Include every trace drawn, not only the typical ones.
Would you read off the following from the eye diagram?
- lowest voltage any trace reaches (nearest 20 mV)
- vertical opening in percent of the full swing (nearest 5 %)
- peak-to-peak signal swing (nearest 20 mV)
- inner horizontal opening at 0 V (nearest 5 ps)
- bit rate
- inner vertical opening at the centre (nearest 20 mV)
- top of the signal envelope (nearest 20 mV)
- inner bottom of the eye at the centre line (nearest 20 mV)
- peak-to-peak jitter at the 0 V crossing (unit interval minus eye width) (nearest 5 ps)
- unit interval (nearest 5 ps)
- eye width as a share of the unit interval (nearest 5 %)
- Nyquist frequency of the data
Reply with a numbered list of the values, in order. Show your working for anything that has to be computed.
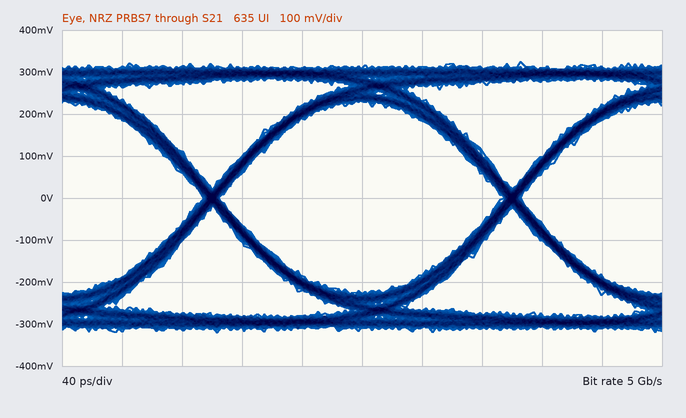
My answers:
1. -320 mV
2. 460 mV / 640 mV ≈ 71.9 %, so 70 % to the nearest 5 %
3. 640 mV
4. 190 ps
5. 5 Gb/s
6. 460 mV
7. 320 mV
8. -220 mV
9. 10 ps
10. 200 ps
11. 190 ps / 200 ps ≈ 95 %
12. 2.5 GHz
